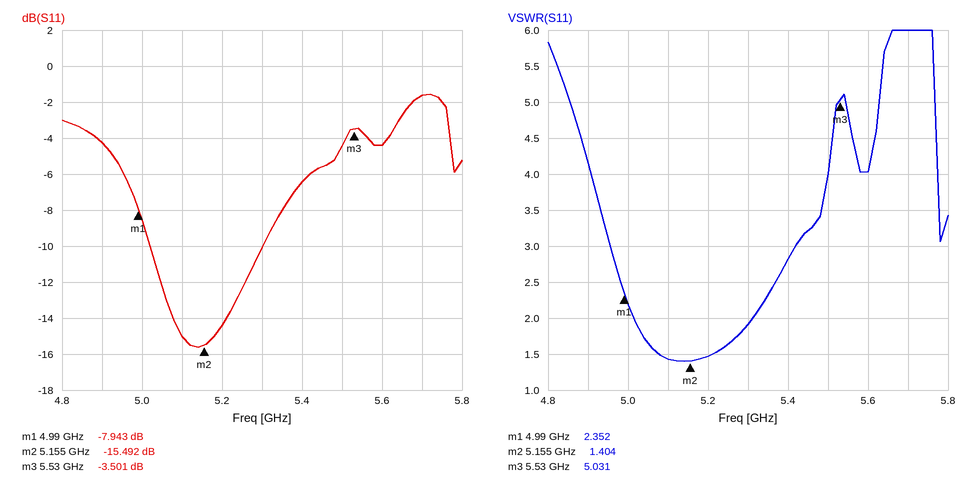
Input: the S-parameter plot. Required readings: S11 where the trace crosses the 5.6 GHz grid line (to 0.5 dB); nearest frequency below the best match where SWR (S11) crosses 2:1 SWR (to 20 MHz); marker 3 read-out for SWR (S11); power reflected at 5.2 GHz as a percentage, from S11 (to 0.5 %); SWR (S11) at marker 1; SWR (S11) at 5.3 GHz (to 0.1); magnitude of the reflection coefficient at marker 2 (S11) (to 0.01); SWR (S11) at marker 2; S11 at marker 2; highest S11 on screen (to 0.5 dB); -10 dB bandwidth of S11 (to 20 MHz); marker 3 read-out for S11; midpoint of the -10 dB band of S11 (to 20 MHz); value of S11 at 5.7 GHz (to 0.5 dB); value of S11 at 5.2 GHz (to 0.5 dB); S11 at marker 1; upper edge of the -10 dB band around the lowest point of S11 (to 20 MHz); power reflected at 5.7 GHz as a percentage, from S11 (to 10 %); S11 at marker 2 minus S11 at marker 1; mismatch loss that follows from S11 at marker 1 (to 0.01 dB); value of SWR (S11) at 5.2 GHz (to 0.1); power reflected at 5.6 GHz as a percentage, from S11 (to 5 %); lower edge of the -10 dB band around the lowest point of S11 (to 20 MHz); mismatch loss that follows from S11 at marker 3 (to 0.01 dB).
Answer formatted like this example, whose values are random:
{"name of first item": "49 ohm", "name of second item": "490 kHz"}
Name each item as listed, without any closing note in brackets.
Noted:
{"S11 where the trace crosses the 5.6 GHz grid line": "-4.5 dB", "nearest frequency below the best match where SWR (S11) crosses 2:1 SWR": "5.02 GHz", "marker 3 read-out for SWR": "5.031", "power reflected at 5.2 GHz as a percentage, from S11": "3.5 %", "SWR (S11) at marker 1": "2.352", "SWR (S11) at 5.3 GHz": "1.9", "magnitude of the reflection coefficient at marker 2 (S11)": "0.17", "SWR (S11) at marker 2": "1.404", "S11 at marker 2": "-15.492 dB", "highest S11 on screen": "-1.5 dB", "-10 dB bandwidth of S11": "280 MHz", "marker 3 read-out for S11": "-3.501 dB", "midpoint of the -10 dB band of S11": "5.16 GHz", "value of S11 at 5.7 GHz": "-1.5 dB", "value of S11 at 5.2 GHz": "-14.5 dB", "S11 at marker 1": "-7.943 dB", "upper edge of the -10 dB band around the lowest point of S11": "5.30 GHz", "power reflected at 5.7 GHz as a percentage, from S11": "70 %", "S11 at marker 2 minus S11 at marker 1": "-7.549 dB", "mismatch loss that follows from S11 at marker 1": "0.76 dB", "value of SWR (S11) at 5.2 GHz": "1.5", "power reflected at 5.6 GHz as a percentage, from S11": "35 %", "lower edge of the -10 dB band around the lowest point of S11": "5.02 GHz", "mismatch loss that follows from S11 at marker 3": "2.57 dB"}
